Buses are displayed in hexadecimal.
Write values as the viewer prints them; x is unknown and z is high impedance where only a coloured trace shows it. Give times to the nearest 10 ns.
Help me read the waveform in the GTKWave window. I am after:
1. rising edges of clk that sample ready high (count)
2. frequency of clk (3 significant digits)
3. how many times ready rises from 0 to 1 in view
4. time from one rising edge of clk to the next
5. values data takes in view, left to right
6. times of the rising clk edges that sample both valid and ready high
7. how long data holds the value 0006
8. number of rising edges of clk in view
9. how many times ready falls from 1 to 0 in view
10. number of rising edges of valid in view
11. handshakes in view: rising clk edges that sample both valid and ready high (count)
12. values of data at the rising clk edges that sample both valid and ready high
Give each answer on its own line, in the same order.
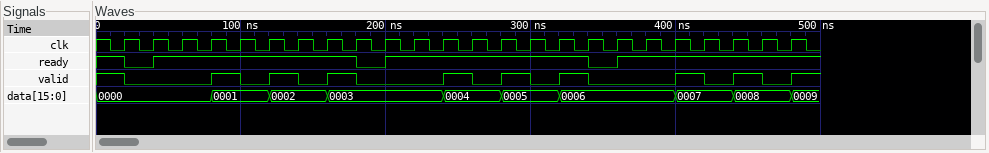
21
50.0 MHz
3
20 ns
0000, 0001, 0002, 0003, 0004, 0005, 0006, 0007, 0008, 0009
20 ns, 100 ns, 140 ns, 180 ns, 260 ns, 300 ns, 340 ns, 420 ns, 460 ns
80 ns
24
3
9
9
0000, 0001, 0002, 0003, 0004, 0005, 0006, 0007, 0008
